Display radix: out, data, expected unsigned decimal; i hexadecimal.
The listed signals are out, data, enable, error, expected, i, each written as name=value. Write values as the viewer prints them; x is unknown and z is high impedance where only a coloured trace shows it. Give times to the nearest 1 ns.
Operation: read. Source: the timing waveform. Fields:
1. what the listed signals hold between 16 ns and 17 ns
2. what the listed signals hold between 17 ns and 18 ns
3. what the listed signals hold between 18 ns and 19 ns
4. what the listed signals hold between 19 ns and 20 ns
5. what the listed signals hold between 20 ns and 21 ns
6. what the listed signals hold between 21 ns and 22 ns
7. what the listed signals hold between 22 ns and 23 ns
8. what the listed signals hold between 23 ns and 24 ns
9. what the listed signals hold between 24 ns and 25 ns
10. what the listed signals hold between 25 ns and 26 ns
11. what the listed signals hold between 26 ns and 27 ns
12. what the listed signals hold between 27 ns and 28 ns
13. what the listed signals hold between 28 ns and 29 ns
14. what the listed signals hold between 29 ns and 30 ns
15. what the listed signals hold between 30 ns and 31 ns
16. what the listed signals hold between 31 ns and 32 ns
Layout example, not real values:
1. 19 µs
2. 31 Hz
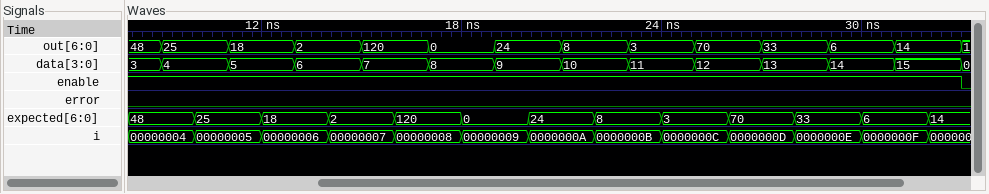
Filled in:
1. out=120, data=7, enable=1, error=0, expected=120, i=00000008
2. out=0, data=8, enable=1, error=0, expected=120, i=00000008
3. out=0, data=8, enable=1, error=0, expected=0, i=00000009
4. out=24, data=9, enable=1, error=0, expected=0, i=00000009
5. out=24, data=9, enable=1, error=0, expected=24, i=0000000A
6. out=8, data=10, enable=1, error=0, expected=24, i=0000000A
7. out=8, data=10, enable=1, error=0, expected=8, i=0000000B
8. out=3, data=11, enable=1, error=0, expected=8, i=0000000B
9. out=3, data=11, enable=1, error=0, expected=3, i=0000000C
10. out=70, data=12, enable=1, error=0, expected=3, i=0000000C
11. out=70, data=12, enable=1, error=0, expected=70, i=0000000D
12. out=33, data=13, enable=1, error=0, expected=70, i=0000000D
13. out=33, data=13, enable=1, error=0, expected=33, i=0000000E
14. out=6, data=14, enable=1, error=0, expected=33, i=0000000E
15. out=6, data=14, enable=1, error=0, expected=6, i=0000000F
16. out=14, data=15, enable=1, error=0, expected=6, i=0000000F
